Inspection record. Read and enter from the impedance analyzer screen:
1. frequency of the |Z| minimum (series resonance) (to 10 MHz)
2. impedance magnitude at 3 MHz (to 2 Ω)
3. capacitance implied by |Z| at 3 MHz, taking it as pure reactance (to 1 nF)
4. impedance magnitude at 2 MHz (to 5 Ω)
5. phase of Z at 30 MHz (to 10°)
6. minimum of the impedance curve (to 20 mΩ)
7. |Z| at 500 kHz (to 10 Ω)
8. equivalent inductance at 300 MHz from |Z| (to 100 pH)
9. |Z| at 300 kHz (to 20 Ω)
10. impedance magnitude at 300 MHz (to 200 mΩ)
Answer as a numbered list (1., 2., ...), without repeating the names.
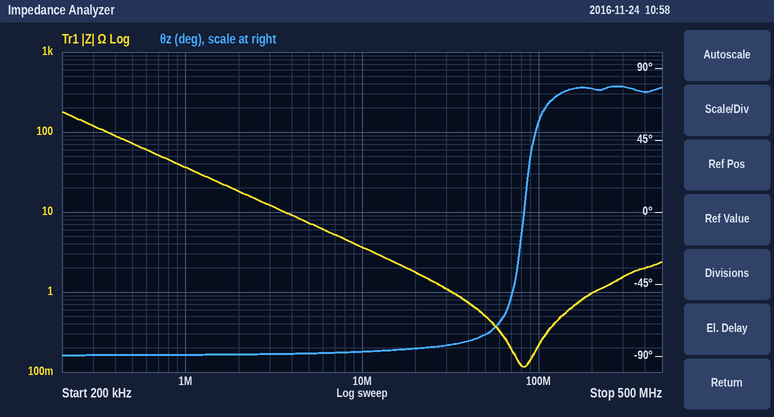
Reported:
1. 80 MHz
2. 12 Ω
3. 4 nF
4. 20 Ω
5. -80°
6. 120 mΩ
7. 70 Ω
8. 800 pH
9. 120 Ω
10. 1.6 Ω
